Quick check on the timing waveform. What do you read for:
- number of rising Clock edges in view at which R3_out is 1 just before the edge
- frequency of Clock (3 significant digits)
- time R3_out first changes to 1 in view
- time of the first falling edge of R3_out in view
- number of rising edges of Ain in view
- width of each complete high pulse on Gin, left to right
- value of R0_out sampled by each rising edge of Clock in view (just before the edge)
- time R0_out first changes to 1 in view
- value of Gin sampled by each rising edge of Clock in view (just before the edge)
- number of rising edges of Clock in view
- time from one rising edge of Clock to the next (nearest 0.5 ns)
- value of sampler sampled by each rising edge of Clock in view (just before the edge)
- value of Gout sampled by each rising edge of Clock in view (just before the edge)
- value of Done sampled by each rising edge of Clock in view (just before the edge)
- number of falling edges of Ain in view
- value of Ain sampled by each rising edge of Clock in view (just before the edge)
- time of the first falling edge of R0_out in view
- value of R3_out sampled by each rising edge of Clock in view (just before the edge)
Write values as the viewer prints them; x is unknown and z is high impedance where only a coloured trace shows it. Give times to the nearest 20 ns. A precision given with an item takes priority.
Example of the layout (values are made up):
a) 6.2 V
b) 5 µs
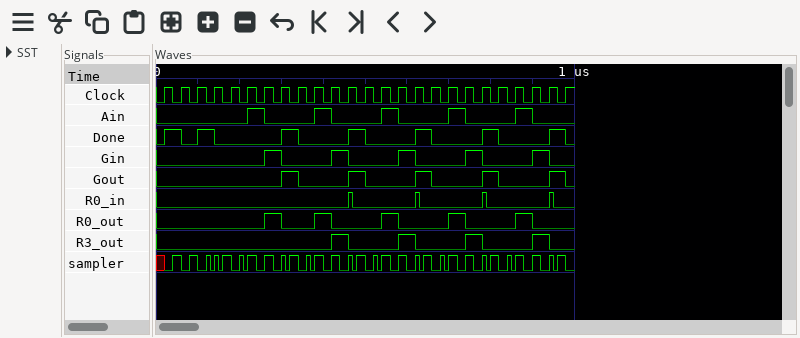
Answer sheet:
a) 4
b) 25.0 MHz
c) 420 ns
d) 460 ns
e) 5
f) 40 ns, 40 ns, 40 ns, 40 ns, 40 ns
g) 0 0 0 0 0 0 0 1 0 0 1 0 0 0 1 0 0 0 1 0 0 0 1 0 0
h) 260 ns
i) 0 0 0 0 0 0 0 1 0 0 0 1 0 0 0 1 0 0 0 1 0 0 0 1 0
j) 25
k) 40 ns
l) x 1 1 0 1 0 0 0 1 0 0 0 1 0 0 0 1 0 0 0 1 0 0 0 1
m) 0 0 0 0 0 0 0 0 1 0 0 0 1 0 0 0 1 0 0 0 1 0 0 0 1
n) 0 1 0 1 0 0 0 0 1 0 0 0 1 0 0 0 1 0 0 0 1 0 0 0 1
o) 5
p) 0 0 0 0 0 0 1 0 0 0 1 0 0 0 1 0 0 0 1 0 0 0 1 0 0
q) 300 ns
r) 0 0 0 0 0 0 0 0 0 0 0 1 0 0 0 1 0 0 0 1 0 0 0 1 0
